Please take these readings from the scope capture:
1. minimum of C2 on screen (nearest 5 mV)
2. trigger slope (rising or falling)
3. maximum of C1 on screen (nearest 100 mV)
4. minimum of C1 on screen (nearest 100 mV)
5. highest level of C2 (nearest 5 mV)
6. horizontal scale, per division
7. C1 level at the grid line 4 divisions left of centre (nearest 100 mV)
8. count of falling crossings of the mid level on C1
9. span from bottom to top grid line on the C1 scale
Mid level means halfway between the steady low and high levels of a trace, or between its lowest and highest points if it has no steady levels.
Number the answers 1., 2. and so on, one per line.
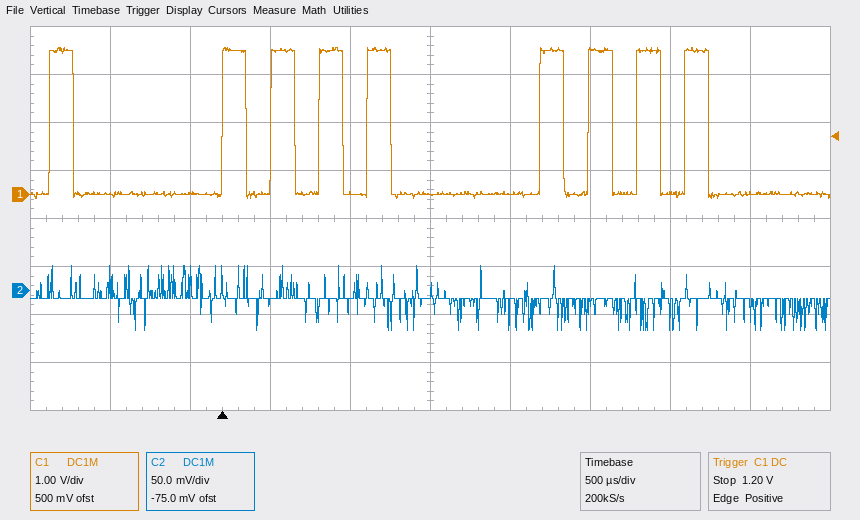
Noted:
1. -40 mV
2. rising
3. 3.1 V
4. -100 mV
5. 25 mV
6. 500 µs
7. 0.0 V
8. 9
9. 8 V
